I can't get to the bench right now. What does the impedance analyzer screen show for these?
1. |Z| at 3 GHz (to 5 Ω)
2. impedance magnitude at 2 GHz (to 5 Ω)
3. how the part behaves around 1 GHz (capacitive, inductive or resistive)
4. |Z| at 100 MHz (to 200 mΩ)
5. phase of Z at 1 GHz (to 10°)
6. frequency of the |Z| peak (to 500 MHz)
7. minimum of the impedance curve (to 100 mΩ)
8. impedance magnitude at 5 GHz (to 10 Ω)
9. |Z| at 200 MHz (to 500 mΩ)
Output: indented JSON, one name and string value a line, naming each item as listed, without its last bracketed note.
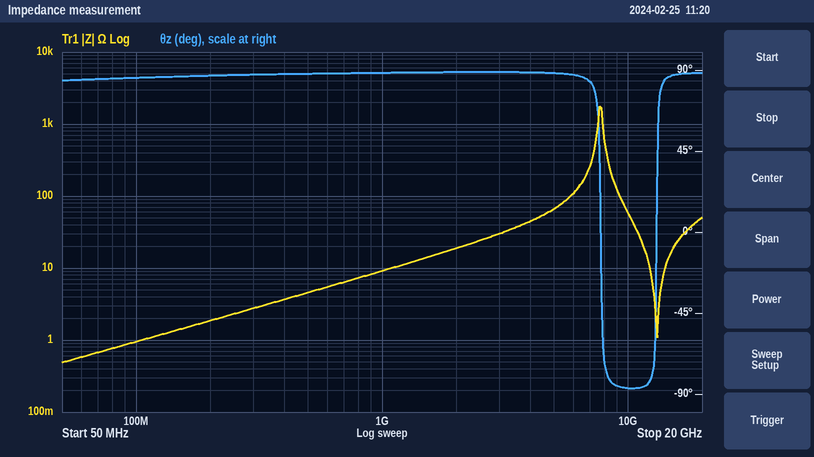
{
  "|Z| at 3 GHz": "30 Ω",
  "impedance magnitude at 2 GHz": "20 Ω",
  "how the part behaves around 1 GHz": "inductive",
  "|Z| at 100 MHz": "1.0 Ω",
  "phase of Z at 1 GHz": "90°",
  "frequency of the |Z| peak": "7.5 GHz",
  "minimum of the impedance curve": "500 mΩ",
  "impedance magnitude at 5 GHz": "70 Ω",
  "|Z| at 200 MHz": "2.0 Ω"
}
